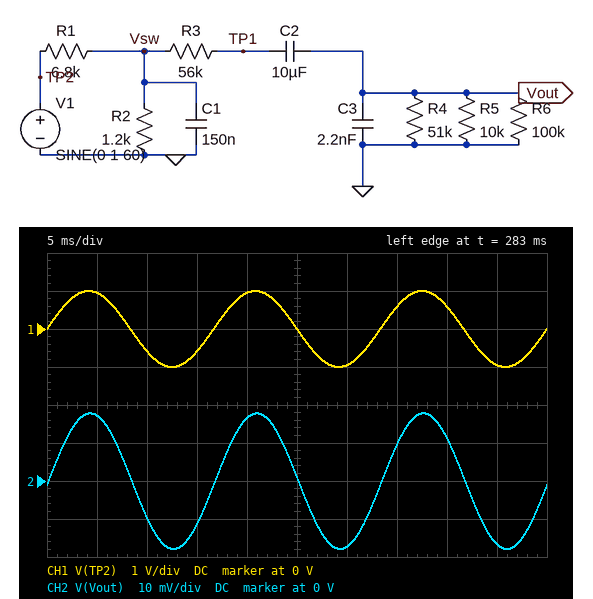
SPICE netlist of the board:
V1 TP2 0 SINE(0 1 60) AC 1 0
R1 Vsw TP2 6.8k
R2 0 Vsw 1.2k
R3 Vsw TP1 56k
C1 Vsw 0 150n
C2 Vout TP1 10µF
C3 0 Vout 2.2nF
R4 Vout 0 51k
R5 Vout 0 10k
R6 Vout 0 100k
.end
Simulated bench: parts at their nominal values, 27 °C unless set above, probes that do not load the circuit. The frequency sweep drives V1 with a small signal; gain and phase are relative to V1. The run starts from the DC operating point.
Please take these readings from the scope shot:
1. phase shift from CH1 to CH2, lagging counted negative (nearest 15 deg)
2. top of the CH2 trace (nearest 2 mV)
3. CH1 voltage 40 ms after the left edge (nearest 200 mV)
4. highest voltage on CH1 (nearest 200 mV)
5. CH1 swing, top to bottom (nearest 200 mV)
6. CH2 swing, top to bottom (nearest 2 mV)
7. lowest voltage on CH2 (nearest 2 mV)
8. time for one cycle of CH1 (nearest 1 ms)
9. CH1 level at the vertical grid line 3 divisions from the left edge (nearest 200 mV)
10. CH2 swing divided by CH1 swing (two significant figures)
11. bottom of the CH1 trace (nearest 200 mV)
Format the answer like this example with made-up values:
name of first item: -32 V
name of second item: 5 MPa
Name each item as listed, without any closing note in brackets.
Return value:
phase shift from CH1 to CH2, lagging counted negative: 0 deg
top of the CH2 trace: 18 mV
CH1 voltage 40 ms after the left edge: 600 mV
highest voltage on CH1: 1.0 V
CH1 swing, top to bottom: 2.0 V
CH2 swing, top to bottom: 36 mV
lowest voltage on CH2: -18 mV
time for one cycle of CH1: 17 ms
CH1 level at the vertical grid line 3 divisions from the left edge: -600 mV
CH2 swing divided by CH1 swing: 0.018
bottom of the CH1 trace: -1.0 V
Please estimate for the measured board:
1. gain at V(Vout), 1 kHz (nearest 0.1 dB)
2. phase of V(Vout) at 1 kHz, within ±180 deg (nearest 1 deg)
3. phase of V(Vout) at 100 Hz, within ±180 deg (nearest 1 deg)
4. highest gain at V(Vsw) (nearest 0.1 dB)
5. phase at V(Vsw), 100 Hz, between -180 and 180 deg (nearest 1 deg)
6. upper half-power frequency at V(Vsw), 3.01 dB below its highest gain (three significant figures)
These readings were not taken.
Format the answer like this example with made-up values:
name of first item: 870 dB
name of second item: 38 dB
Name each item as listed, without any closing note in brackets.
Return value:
gain at V(Vout), 1 kHz: -37.8 dB
phase of V(Vout) at 1 kHz, within ±180 deg: -49 deg
phase of V(Vout) at 100 Hz, within ±180 deg: -6 deg
highest gain at V(Vsw): -16.5 dB
phase at V(Vsw), 100 Hz, between -180 and 180 deg: -5 deg
upper half-power frequency at V(Vsw), 3.01 dB below its highest gain: 1.02 kHz
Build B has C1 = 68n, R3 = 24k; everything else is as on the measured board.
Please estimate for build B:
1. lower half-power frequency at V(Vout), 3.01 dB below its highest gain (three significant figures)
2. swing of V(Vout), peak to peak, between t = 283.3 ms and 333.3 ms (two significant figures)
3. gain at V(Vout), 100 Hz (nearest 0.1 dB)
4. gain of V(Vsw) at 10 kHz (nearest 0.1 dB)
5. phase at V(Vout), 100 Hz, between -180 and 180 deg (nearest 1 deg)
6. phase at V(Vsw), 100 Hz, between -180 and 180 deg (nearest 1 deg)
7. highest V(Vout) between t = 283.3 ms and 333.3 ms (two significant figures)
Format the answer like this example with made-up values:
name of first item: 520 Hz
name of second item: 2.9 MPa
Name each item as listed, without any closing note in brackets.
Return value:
lower half-power frequency at V(Vout), 3.01 dB below its highest gain: 486 mHz
swing of V(Vout), peak to peak, between t = 283.3 ms and 333.3 ms: 71 mV
gain at V(Vout), 100 Hz: -29.0 dB
gain of V(Vsw) at 10 kHz: -29.5 dB
phase at V(Vout), 100 Hz, between -180 and 180 deg: -3 deg
phase at V(Vsw), 100 Hz, between -180 and 180 deg: -2 deg
highest V(Vout) between t = 283.3 ms and 333.3 ms: 35 mV
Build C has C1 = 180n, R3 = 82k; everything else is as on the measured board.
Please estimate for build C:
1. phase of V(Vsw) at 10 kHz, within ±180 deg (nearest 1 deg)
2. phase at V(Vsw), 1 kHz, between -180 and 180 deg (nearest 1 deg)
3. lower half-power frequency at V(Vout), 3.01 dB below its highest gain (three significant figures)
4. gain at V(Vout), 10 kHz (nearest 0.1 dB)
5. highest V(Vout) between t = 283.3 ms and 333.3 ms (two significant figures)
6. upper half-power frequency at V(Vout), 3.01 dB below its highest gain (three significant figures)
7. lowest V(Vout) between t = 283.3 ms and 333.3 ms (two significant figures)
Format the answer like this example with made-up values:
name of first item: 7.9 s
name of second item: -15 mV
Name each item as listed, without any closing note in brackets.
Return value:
phase of V(Vsw) at 10 kHz, within ±180 deg: -85 deg
phase at V(Vsw), 1 kHz, between -180 and 180 deg: -49 deg
lower half-power frequency at V(Vout), 3.01 dB below its highest gain: 175 mHz
gain at V(Vout), 10 kHz: -62.0 dB
highest V(Vout) between t = 283.3 ms and 333.3 ms: 13 mV
upper half-power frequency at V(Vout), 3.01 dB below its highest gain: 871 Hz
lowest V(Vout) between t = 283.3 ms and 333.3 ms: -13 mV
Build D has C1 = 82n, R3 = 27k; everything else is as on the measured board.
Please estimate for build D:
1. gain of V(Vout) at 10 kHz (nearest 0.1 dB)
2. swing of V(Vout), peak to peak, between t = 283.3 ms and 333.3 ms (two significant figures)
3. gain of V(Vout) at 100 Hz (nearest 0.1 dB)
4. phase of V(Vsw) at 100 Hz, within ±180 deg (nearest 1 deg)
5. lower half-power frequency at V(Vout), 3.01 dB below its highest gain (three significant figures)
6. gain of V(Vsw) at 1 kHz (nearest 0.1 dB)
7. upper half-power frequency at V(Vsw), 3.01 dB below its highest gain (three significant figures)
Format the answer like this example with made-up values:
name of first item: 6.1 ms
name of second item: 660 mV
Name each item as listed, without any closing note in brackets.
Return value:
gain of V(Vout) at 10 kHz: -46.4 dB
swing of V(Vout), peak to peak, between t = 283.3 ms and 333.3 ms: 65 mV
gain of V(Vout) at 100 Hz: -29.8 dB
phase of V(Vsw) at 100 Hz, within ±180 deg: -3 deg
lower half-power frequency at V(Vout), 3.01 dB below its highest gain: 445 mHz
gain of V(Vsw) at 1 kHz: -17.7 dB
upper half-power frequency at V(Vsw), 3.01 dB below its highest gain: 1.84 kHz
